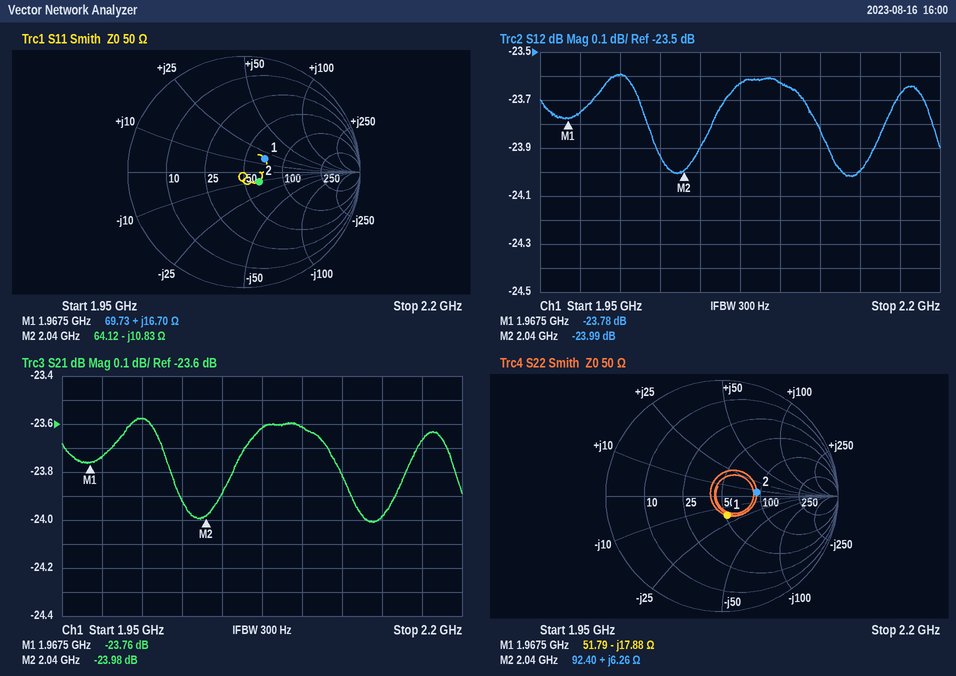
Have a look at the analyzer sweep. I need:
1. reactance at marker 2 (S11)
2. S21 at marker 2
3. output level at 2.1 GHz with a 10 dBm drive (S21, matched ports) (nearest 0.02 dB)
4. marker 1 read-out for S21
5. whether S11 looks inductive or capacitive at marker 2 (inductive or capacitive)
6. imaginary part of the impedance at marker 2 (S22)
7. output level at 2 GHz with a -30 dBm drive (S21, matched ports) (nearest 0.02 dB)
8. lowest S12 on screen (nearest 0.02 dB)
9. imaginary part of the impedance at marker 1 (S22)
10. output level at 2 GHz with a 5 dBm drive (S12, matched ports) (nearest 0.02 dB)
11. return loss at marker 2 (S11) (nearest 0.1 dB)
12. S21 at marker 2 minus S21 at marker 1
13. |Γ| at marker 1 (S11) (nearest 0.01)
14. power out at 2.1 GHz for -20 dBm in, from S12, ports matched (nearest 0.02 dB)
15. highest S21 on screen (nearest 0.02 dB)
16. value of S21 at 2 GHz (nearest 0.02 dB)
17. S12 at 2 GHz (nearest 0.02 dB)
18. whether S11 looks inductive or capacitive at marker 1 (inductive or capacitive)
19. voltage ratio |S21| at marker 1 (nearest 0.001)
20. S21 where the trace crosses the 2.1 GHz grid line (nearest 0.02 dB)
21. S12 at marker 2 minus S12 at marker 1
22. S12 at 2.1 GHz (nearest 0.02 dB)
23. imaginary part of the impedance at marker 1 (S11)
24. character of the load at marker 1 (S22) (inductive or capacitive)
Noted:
-10.83 Ω
-23.98 dB
-13.62 dBm
-23.76 dB
capacitive
+6.26 Ω
-53.58 dBm
-24.02 dB
-17.88 Ω
-18.60 dBm
16.2 dB
-0.22 dB
0.21
-43.62 dBm
-23.58 dB
-23.58 dB
-23.60 dB
inductive
0.065
-23.62 dB
-0.21 dB
-23.62 dB
+16.70 Ω
capacitive
